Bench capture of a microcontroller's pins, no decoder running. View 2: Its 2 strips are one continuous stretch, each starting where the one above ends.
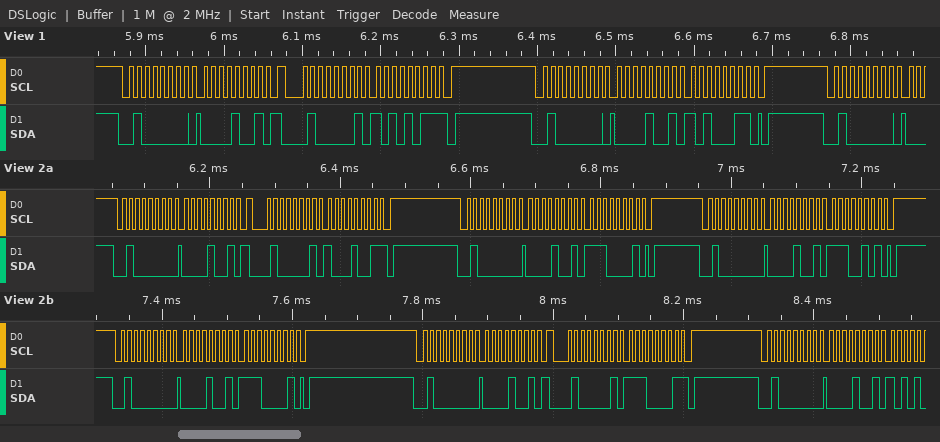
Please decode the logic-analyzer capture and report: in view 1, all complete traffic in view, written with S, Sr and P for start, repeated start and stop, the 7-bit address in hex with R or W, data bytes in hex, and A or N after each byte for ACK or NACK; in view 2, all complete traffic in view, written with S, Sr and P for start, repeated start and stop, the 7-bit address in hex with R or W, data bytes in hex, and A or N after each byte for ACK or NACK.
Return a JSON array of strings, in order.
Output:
["S 20W A 09 A Sr 20R A AB N P S 20W A 09 A A3 A P S 20W A", "S 20W A 09 A Sr 20R A 89 N P S 20W A 09 A E1 A P S 20W A 09 A E5 A P S 20W A 09 A E1 A P S 20W A 09 A Sr 20R A E1 N P S 20W A 09 A"]
